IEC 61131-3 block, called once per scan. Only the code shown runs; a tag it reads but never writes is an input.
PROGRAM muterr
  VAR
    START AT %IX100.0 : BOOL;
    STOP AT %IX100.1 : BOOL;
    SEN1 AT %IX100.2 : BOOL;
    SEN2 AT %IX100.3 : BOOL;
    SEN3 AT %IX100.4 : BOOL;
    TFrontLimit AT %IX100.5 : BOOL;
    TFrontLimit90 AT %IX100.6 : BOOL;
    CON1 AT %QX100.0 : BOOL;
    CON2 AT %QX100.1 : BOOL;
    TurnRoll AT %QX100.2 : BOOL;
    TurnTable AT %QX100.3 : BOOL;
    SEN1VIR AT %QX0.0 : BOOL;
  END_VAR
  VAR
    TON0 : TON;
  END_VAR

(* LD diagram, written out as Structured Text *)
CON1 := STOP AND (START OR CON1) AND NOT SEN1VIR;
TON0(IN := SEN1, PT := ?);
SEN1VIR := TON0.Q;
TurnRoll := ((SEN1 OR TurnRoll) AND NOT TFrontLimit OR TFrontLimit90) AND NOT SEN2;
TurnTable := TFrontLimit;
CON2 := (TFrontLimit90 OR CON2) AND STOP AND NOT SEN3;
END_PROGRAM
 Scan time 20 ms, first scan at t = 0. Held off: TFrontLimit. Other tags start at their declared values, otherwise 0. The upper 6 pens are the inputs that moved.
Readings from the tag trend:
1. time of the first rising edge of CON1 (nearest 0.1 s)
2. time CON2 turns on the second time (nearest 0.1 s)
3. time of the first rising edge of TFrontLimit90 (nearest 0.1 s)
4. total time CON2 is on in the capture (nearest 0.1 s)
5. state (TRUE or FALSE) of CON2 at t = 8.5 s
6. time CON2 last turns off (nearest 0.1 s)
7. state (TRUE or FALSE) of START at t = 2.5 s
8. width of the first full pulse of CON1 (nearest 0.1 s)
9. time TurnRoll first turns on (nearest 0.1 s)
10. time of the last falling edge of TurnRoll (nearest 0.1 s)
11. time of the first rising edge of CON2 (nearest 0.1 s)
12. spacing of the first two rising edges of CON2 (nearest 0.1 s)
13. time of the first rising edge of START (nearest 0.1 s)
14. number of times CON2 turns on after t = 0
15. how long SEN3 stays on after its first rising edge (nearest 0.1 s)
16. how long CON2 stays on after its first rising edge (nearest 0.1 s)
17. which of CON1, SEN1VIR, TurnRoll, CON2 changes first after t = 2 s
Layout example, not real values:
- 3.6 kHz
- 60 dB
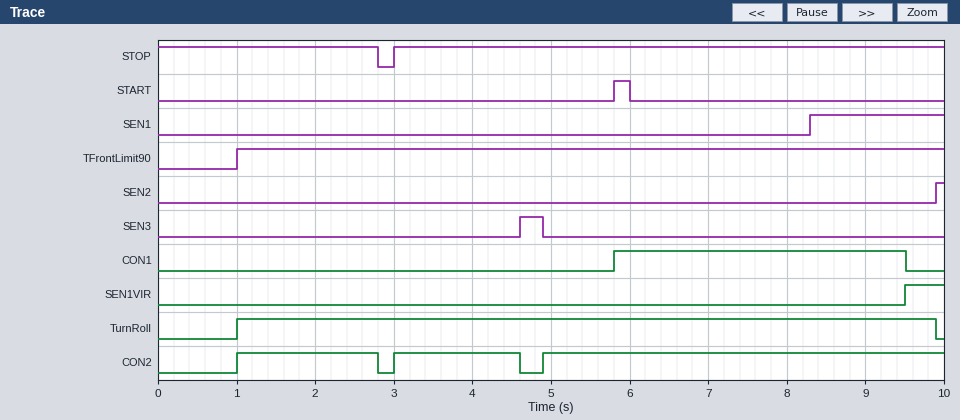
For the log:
- 5.8 s
- 3.0 s
- 1.0 s
- 8.5 s
- TRUE
- 4.6 s
- FALSE
- 3.7 s
- 1.0 s
- 9.9 s
- 1.0 s
- 2.0 s
- 5.8 s
- 3
- 0.3 s
- 1.8 s
- CON2
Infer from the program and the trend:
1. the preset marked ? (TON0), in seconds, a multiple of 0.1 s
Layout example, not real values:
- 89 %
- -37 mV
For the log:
- 1.2 s
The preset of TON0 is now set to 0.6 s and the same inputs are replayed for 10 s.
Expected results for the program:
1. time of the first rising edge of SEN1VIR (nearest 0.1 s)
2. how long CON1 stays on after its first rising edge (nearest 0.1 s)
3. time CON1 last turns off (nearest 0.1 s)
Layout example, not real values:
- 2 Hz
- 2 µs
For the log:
- 8.9 s
- 3.1 s
- 8.9 s
